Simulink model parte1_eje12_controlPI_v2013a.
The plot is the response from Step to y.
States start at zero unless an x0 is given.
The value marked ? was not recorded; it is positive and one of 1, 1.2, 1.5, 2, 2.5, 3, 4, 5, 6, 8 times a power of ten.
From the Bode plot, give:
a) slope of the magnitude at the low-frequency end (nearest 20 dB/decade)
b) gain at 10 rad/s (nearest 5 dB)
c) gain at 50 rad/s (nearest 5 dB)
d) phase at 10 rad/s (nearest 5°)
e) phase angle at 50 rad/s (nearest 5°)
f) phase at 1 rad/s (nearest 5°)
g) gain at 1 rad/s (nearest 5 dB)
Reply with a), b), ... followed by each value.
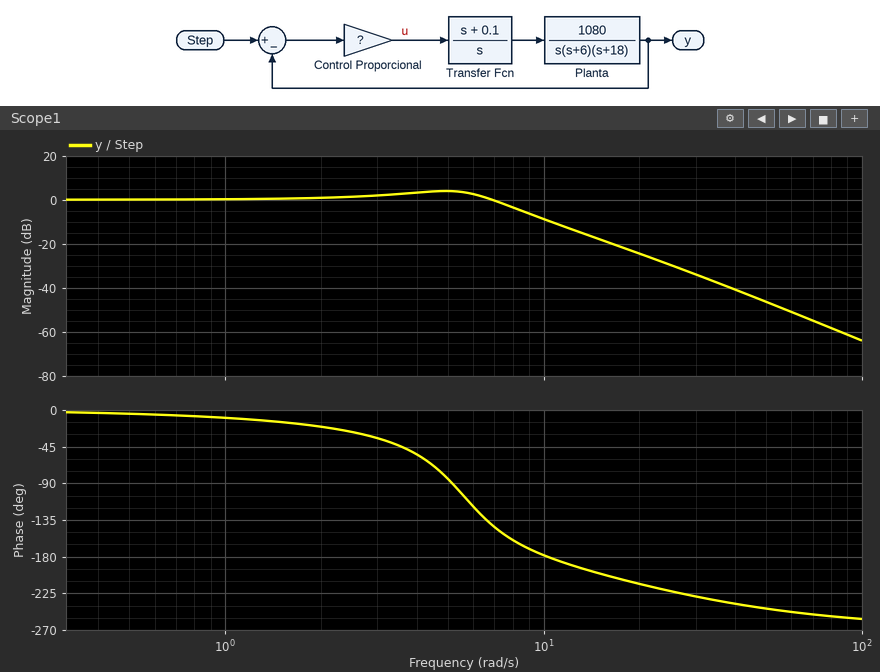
a) 0 dB/decade
b) -10 dB
c) -45 dB
d) -180°
e) -245°
f) -10°
g) 0 dB
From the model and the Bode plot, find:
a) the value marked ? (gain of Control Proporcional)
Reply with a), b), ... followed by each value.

a) 0.6
